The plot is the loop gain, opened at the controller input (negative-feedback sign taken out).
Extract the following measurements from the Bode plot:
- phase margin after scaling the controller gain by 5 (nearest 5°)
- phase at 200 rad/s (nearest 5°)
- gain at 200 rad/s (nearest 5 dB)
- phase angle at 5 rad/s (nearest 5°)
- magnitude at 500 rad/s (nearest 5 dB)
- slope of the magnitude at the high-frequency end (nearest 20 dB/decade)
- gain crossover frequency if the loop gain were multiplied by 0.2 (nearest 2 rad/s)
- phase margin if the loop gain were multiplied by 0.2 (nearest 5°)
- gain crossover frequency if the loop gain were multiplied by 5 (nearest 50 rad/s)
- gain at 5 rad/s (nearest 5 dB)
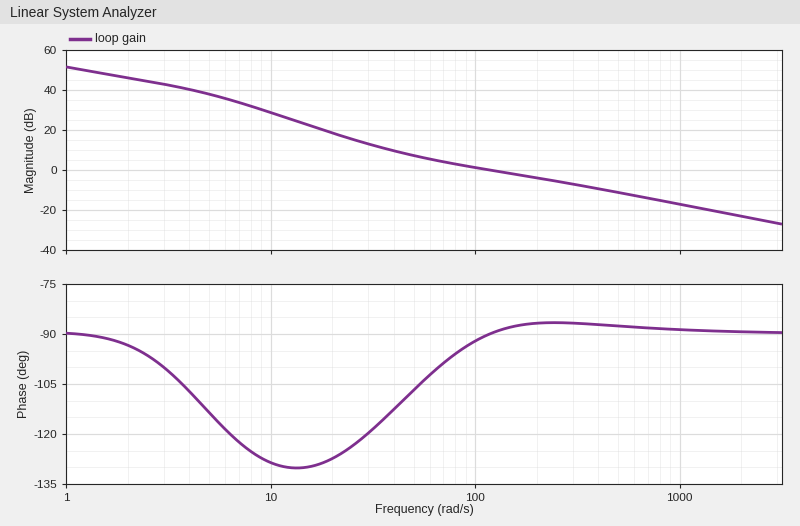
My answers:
90°
-85°
-5 dB
-115°
-10 dB
-20 dB/decade
28 rad/s
60°
700 rad/s
40 dB
